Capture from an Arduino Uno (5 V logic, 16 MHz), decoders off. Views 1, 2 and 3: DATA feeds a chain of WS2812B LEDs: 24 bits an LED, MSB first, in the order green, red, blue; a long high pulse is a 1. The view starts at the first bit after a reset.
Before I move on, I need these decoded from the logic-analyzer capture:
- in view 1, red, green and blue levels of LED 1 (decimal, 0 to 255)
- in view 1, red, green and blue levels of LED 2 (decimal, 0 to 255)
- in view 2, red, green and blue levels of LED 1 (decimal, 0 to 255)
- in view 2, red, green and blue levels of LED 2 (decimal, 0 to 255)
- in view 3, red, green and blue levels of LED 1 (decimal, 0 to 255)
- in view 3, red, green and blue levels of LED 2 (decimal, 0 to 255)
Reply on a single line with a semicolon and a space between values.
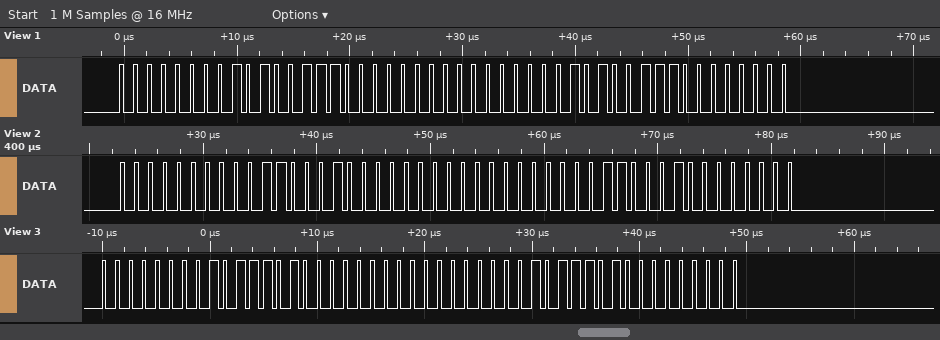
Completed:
167, 0, 0; 167, 0, 0; 49, 0, 0; 49, 0, 0; 186, 0, 0; 186, 0, 0
